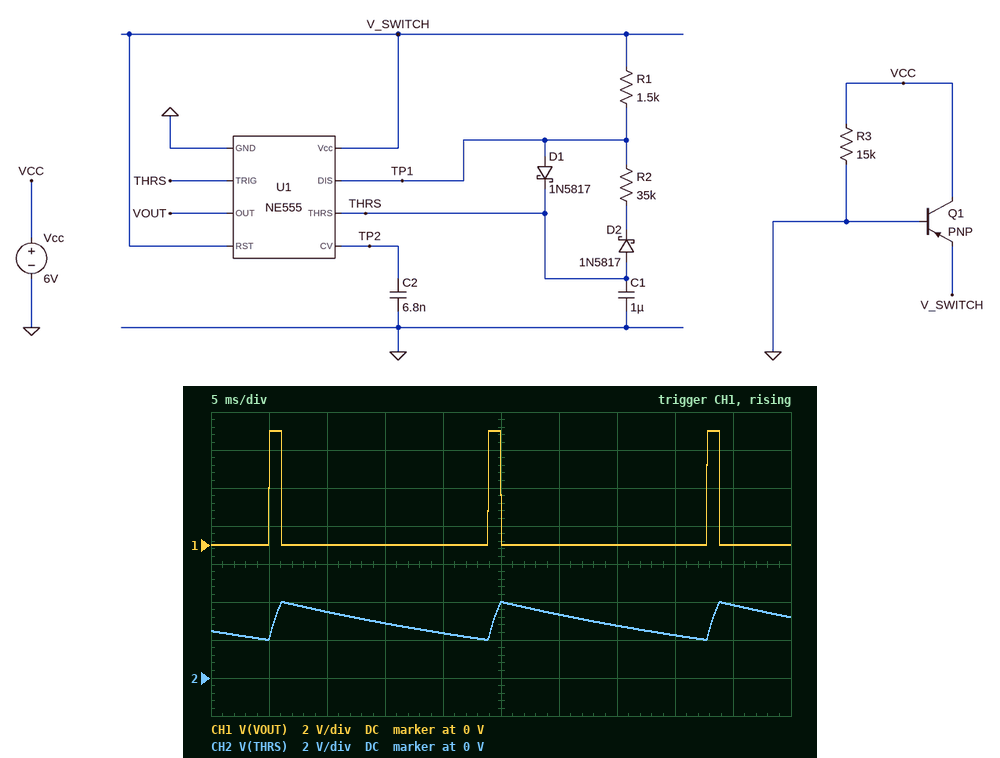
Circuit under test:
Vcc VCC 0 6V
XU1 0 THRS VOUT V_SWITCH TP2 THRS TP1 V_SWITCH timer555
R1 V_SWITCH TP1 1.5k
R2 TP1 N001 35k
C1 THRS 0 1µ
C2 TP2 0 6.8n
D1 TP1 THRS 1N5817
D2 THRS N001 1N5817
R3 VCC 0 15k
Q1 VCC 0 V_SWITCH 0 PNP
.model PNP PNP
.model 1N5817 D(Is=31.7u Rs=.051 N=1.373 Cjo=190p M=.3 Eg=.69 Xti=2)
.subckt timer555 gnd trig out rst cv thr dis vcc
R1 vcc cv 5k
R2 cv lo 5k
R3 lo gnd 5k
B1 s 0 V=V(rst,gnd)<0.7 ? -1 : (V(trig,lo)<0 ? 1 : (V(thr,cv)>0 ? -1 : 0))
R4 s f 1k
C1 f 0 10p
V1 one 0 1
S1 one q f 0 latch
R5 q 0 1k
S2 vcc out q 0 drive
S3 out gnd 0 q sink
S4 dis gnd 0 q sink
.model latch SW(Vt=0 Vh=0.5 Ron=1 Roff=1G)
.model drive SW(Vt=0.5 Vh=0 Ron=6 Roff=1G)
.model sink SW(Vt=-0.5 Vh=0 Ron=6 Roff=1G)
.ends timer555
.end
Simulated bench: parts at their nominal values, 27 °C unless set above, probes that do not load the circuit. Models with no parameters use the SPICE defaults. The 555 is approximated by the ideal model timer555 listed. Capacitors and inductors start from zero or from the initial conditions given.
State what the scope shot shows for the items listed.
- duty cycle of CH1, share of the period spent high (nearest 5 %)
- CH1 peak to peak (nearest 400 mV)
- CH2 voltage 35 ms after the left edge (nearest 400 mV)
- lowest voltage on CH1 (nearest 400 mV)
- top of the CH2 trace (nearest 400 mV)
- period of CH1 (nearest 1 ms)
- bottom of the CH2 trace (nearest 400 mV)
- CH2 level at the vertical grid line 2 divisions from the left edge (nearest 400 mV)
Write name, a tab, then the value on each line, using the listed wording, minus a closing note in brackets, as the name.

duty cycle of CH1, share of the period spent high	5 %
CH1 peak to peak	6.0 V
CH2 voltage 35 ms after the left edge	2.8 V
lowest voltage on CH1	0 V
top of the CH2 trace	4.0 V
period of CH1	19 ms
bottom of the CH2 trace	2.0 V
CH2 level at the vertical grid line 2 divisions from the left edge	3.6 V
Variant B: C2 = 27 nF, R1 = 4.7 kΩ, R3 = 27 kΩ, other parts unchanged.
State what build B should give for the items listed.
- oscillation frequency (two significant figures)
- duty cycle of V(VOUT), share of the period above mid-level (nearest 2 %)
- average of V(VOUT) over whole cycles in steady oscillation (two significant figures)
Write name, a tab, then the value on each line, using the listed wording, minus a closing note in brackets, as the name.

oscillation frequency	48 Hz
duty cycle of V(VOUT), share of the period above mid-level	16 %
average of V(VOUT) over whole cycles in steady oscillation	970 mV
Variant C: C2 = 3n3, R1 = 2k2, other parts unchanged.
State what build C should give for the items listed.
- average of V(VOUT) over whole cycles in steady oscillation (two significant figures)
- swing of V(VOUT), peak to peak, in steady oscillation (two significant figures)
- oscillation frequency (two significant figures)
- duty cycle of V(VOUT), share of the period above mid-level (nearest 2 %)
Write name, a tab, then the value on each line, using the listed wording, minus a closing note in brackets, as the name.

average of V(VOUT) over whole cycles in steady oscillation	500 mV
swing of V(VOUT), peak to peak, in steady oscillation	6.0 V
oscillation frequency	52 Hz
duty cycle of V(VOUT), share of the period above mid-level	8 %
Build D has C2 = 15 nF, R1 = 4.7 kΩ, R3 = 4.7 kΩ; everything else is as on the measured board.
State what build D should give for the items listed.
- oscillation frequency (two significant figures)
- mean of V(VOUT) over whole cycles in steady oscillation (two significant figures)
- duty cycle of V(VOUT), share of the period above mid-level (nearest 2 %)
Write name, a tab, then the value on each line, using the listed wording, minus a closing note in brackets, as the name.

oscillation frequency	48 Hz
mean of V(VOUT) over whole cycles in steady oscillation	970 mV
duty cycle of V(VOUT), share of the period above mid-level	16 %
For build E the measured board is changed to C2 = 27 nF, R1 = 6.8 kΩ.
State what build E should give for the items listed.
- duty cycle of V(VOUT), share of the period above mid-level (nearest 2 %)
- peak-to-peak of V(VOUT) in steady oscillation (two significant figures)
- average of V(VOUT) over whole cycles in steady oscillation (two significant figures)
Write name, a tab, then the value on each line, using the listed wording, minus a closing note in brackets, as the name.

duty cycle of V(VOUT), share of the period above mid-level	22 %
peak-to-peak of V(VOUT) in steady oscillation	6.0 V
average of V(VOUT) over whole cycles in steady oscillation	1.3 V
